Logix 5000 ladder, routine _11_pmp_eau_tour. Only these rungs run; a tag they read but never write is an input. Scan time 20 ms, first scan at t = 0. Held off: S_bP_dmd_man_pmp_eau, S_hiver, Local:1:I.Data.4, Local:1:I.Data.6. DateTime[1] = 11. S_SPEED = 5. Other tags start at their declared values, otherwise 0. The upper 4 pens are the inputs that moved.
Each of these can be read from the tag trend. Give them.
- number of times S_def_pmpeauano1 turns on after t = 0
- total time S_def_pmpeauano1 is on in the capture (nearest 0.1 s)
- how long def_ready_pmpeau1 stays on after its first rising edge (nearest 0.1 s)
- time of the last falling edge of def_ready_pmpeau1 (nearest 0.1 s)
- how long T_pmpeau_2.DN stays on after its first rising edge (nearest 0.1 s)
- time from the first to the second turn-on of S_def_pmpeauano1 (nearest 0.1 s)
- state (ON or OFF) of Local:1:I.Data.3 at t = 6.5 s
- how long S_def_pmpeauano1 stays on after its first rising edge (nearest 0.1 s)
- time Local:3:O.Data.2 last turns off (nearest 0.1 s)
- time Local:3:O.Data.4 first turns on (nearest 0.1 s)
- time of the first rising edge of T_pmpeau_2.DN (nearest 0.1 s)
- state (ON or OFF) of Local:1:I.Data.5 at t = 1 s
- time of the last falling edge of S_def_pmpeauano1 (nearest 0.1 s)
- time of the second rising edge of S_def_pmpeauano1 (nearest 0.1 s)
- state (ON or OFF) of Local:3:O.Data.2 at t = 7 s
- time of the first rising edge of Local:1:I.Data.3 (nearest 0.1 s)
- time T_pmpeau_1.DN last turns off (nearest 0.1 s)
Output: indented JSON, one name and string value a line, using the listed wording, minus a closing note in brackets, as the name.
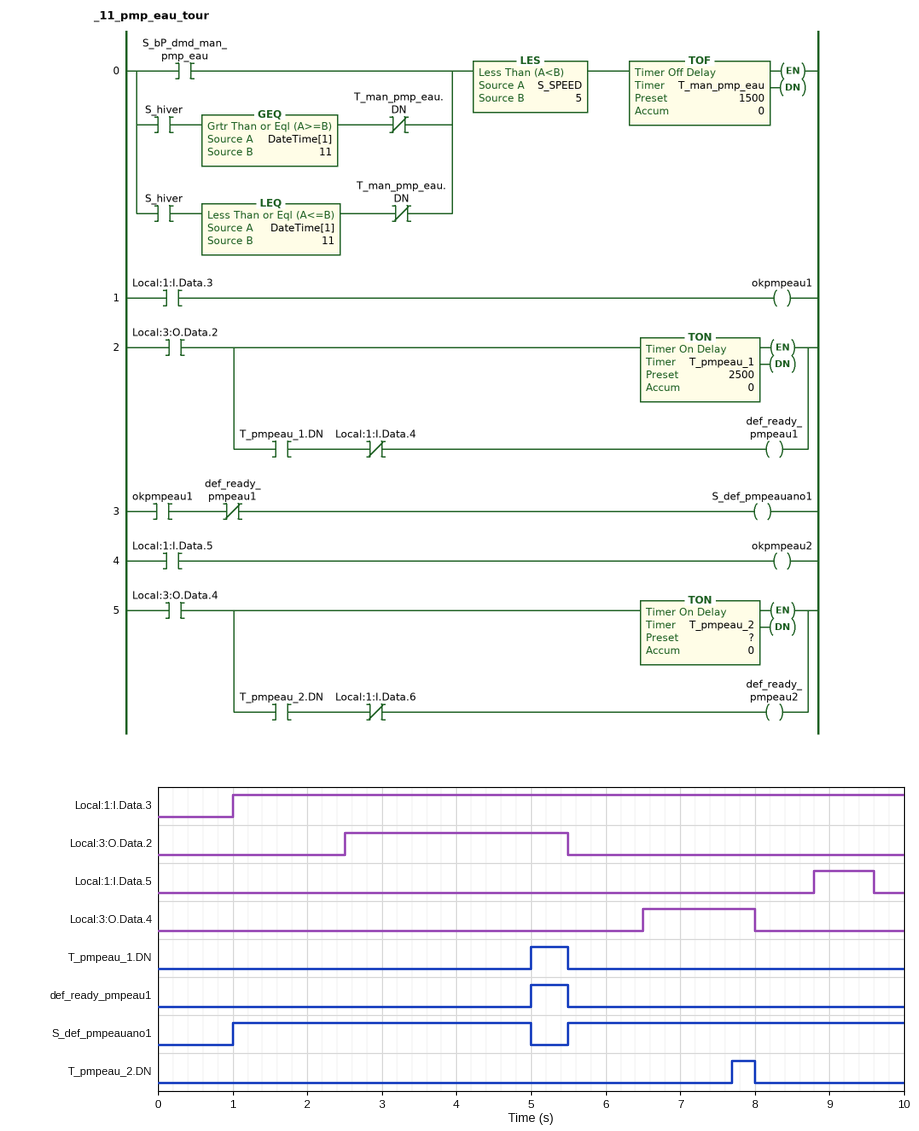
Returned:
{
  "number of times S_def_pmpeauano1 turns on after t = 0": "2",
  "total time S_def_pmpeauano1 is on in the capture": "8.5 s",
  "how long def_ready_pmpeau1 stays on after its first rising edge": "0.5 s",
  "time of the last falling edge of def_ready_pmpeau1": "5.5 s",
  "how long T_pmpeau_2.DN stays on after its first rising edge": "0.3 s",
  "time from the first to the second turn-on of S_def_pmpeauano1": "4.5 s",
  "state (ON or OFF) of Local:1:I.Data.3 at t = 6.5 s": "ON",
  "how long S_def_pmpeauano1 stays on after its first rising edge": "4.0 s",
  "time Local:3:O.Data.2 last turns off": "5.5 s",
  "time Local:3:O.Data.4 first turns on": "6.5 s",
  "time of the first rising edge of T_pmpeau_2.DN": "7.7 s",
  "state (ON or OFF) of Local:1:I.Data.5 at t = 1 s": "OFF",
  "time of the last falling edge of S_def_pmpeauano1": "5.0 s",
  "time of the second rising edge of S_def_pmpeauano1": "5.5 s",
  "state (ON or OFF) of Local:3:O.Data.2 at t = 7 s": "OFF",
  "time of the first rising edge of Local:1:I.Data.3": "1.0 s",
  "time T_pmpeau_1.DN last turns off": "5.5 s"
}
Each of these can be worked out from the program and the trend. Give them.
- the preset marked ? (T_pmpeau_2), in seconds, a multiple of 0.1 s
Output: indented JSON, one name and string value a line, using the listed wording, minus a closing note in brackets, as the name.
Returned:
{
  "the preset marked ? (T_pmpeau_2), in seconds, a multiple of 0.1 s": "1.2 s"
}
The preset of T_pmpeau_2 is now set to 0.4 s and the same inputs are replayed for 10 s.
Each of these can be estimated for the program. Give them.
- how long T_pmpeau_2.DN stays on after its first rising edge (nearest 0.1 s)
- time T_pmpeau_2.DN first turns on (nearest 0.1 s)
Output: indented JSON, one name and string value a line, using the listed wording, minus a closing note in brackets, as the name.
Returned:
{
  "how long T_pmpeau_2.DN stays on after its first rising edge": "1.1 s",
  "time T_pmpeau_2.DN first turns on": "6.9 s"
}
